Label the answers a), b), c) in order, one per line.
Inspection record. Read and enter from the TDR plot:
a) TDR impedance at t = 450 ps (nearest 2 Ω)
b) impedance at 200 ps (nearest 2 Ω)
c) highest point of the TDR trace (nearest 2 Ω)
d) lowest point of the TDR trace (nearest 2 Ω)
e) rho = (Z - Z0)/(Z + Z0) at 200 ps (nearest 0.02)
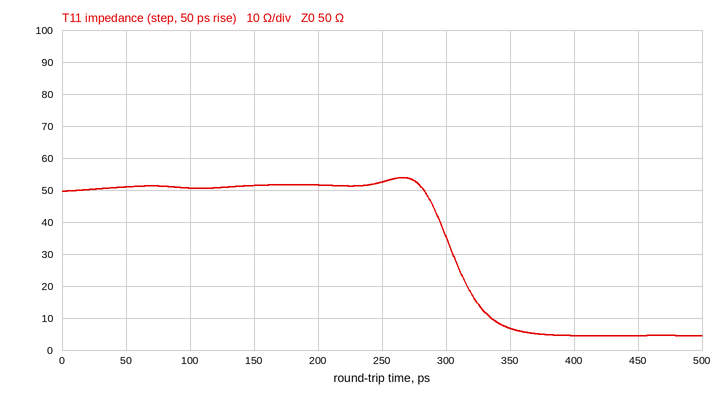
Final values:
a) 4 Ω
b) 52 Ω
c) 54 Ω
d) 4 Ω
e) +0.02
